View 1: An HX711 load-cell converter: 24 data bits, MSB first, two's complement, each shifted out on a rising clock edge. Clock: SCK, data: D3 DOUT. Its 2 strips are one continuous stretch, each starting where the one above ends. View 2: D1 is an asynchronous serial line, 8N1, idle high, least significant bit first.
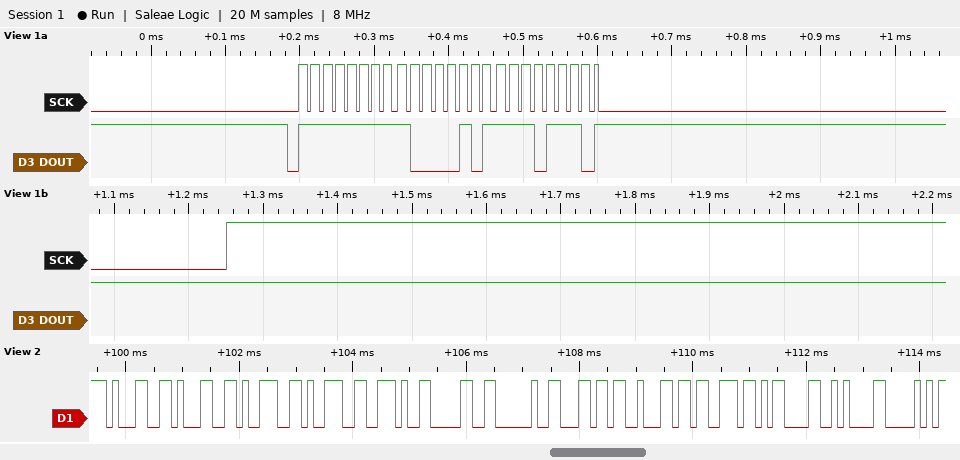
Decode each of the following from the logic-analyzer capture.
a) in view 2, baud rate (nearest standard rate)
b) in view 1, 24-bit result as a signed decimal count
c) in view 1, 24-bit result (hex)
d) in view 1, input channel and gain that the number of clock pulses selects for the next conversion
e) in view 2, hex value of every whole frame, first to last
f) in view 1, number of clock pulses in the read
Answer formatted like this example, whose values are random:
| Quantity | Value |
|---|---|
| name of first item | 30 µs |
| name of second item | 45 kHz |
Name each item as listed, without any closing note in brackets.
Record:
| Quantity | Value |
|---|---|
| in view 2, baud rate | 9600 baud |
| in view 1, 24-bit result as a signed decimal count | -31250 |
| in view 1, 24-bit result | 0xFF85EE |
| in view 1, input channel and gain that the number of clock pulses selects for the next conversion | channel B, gain 32 |
| in view 2, hex value of every whole frame, first to last | 0x31 0x31 0x39 0x39 0x2E 0x30 0x20 0x6C 0x62 0x73 0x0D 0x0A 0x50 |
| in view 1, number of clock pulses in the read | 26 |
